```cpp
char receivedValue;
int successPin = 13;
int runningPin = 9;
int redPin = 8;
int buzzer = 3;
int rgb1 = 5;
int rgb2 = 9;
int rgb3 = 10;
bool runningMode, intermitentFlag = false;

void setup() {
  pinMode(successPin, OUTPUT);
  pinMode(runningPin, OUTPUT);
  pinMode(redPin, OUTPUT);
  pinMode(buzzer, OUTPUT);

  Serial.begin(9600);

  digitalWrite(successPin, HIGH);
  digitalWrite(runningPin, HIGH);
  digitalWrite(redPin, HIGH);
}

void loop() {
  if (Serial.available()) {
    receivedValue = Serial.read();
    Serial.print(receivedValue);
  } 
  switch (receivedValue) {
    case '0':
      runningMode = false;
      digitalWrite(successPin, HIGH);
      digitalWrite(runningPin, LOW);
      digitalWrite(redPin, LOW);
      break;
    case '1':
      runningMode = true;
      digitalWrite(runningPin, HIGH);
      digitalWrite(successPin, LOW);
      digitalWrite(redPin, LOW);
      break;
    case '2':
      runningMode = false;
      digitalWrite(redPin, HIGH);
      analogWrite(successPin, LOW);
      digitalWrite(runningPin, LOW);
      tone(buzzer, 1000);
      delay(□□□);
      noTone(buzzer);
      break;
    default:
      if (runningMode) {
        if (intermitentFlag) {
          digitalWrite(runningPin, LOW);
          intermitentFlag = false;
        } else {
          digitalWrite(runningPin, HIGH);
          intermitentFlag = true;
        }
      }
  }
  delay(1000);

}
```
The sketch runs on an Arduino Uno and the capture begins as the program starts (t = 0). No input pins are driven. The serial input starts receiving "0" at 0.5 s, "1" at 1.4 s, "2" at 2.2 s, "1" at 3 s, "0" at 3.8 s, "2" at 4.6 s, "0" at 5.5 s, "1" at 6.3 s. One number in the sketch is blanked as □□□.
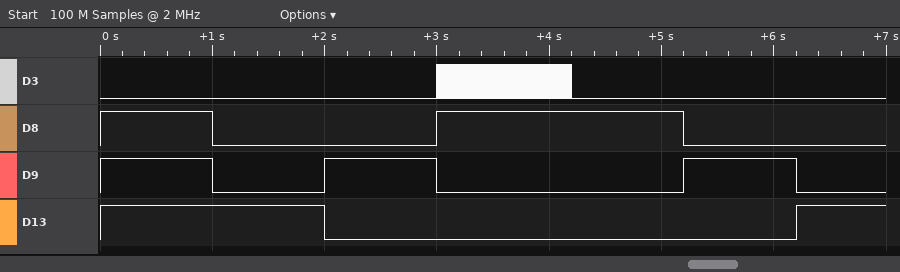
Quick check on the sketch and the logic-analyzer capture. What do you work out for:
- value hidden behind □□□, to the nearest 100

1200
